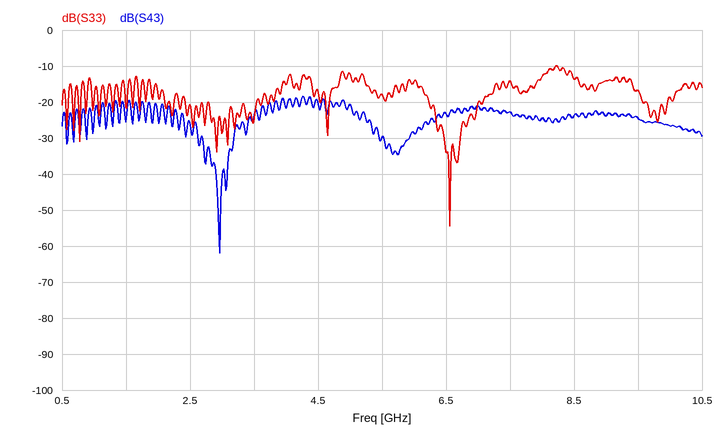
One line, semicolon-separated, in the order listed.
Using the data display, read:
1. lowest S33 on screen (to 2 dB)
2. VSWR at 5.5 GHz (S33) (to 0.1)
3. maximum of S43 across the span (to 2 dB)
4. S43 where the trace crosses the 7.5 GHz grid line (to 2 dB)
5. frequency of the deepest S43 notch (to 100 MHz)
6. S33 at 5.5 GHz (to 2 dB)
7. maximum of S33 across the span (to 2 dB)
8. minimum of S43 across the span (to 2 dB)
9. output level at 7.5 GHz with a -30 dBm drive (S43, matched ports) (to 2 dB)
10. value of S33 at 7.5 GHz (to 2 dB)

-54 dB; 1.3; -18 dB; -22 dB; 3.0 GHz; -18 dB; -10 dB; -62 dB; -52 dBm; -14 dB
